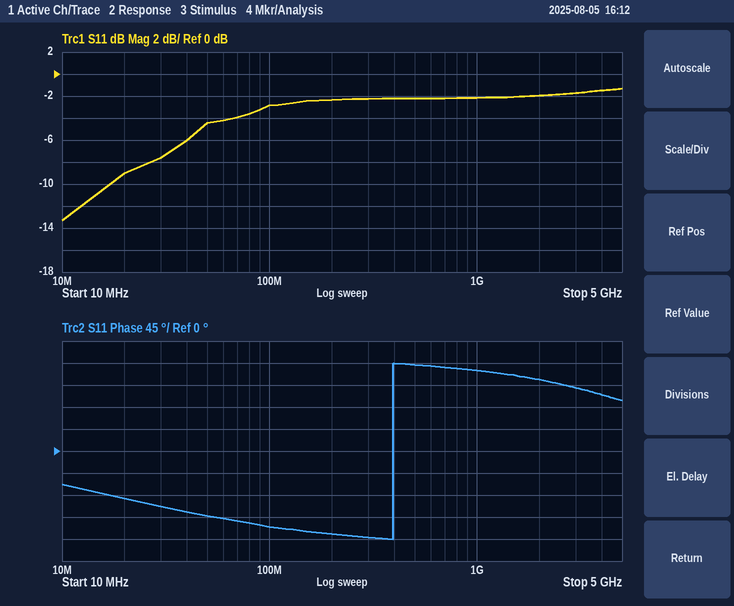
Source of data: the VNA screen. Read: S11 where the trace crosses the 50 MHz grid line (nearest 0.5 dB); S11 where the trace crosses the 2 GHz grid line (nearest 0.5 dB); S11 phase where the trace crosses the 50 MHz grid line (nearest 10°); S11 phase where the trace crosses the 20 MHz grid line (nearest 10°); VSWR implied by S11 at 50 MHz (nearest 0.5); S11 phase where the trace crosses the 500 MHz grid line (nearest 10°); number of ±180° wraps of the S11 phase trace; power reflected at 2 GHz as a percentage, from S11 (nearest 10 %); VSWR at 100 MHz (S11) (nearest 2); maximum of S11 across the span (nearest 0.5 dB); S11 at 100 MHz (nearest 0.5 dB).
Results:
-4.5 dB
-2.0 dB
-130°
-100°
4.0
180°
1
60 %
6
-1.5 dB
-3.0 dB
